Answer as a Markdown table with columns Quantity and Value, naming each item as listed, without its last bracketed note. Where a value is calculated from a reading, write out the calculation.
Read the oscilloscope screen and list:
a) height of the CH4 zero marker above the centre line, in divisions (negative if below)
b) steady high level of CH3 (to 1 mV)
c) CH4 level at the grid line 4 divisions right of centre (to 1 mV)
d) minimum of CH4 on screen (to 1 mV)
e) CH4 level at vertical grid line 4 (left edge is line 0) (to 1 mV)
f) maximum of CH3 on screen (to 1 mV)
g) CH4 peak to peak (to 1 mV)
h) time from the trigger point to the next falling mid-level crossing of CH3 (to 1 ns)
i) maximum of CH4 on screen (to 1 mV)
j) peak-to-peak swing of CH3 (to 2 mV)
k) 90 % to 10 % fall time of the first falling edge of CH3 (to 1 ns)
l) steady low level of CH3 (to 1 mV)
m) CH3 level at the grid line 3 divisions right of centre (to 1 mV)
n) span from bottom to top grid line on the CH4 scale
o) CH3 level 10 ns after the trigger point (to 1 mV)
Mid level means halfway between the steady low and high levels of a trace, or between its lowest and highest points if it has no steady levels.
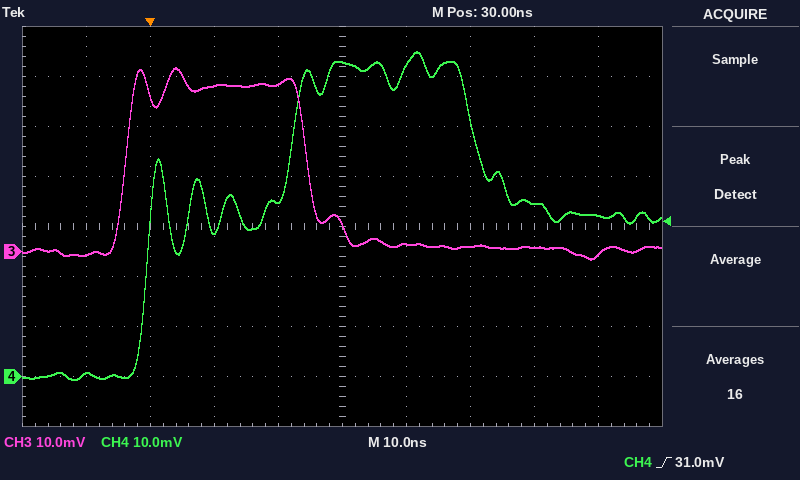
| Quantity | Value |
|---|---|
| height of the CH4 zero marker above the centre line, in divisions | -3.0 div |
| steady high level of CH3 | 33 mV |
| CH4 level at the grid line 4 divisions right of centre | 32 mV |
| minimum of CH4 on screen | -1 mV |
| CH4 level at vertical grid line 4 (left edge is line 0) | 35 mV |
| maximum of CH3 on screen | 37 mV |
| CH4 peak to peak | 65 mV − (-1 mV) = 66 mV |
| time from the trigger point to the next falling mid-level crossing of CH3 | 25 ns |
| maximum of CH4 on screen | 65 mV |
| peak-to-peak swing of CH3 | 38 mV |
| 90 % to 10 % fall time of the first falling edge of CH3 | 7 ns |
| steady low level of CH3 | 1 mV |
| CH3 level at the grid line 3 divisions right of centre | 1 mV |
| span from bottom to top grid line on the CH4 scale | 80 mV |
| CH3 level 10 ns after the trigger point | 33 mV |
